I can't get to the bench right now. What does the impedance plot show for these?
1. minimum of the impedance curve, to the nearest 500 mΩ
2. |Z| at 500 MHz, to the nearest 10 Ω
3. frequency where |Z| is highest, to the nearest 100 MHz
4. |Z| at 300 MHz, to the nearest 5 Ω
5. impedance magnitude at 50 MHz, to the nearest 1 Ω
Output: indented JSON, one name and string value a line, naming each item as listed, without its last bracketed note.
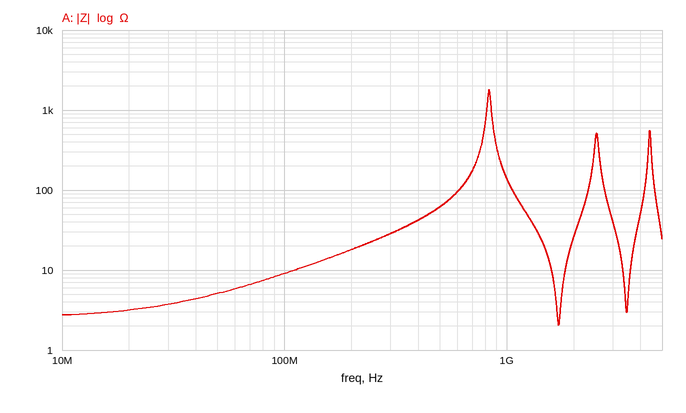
{
  "minimum of the impedance curve, to the nearest 500 mΩ": "2.0 Ω",
  "|Z| at 500 MHz, to the nearest 10 Ω": "60 Ω",
  "frequency where |Z| is highest, to the nearest 100 MHz": "800 MHz",
  "|Z| at 300 MHz, to the nearest 5 Ω": "30 Ω",
  "impedance magnitude at 50 MHz, to the nearest 1 Ω": "5 Ω"
}
